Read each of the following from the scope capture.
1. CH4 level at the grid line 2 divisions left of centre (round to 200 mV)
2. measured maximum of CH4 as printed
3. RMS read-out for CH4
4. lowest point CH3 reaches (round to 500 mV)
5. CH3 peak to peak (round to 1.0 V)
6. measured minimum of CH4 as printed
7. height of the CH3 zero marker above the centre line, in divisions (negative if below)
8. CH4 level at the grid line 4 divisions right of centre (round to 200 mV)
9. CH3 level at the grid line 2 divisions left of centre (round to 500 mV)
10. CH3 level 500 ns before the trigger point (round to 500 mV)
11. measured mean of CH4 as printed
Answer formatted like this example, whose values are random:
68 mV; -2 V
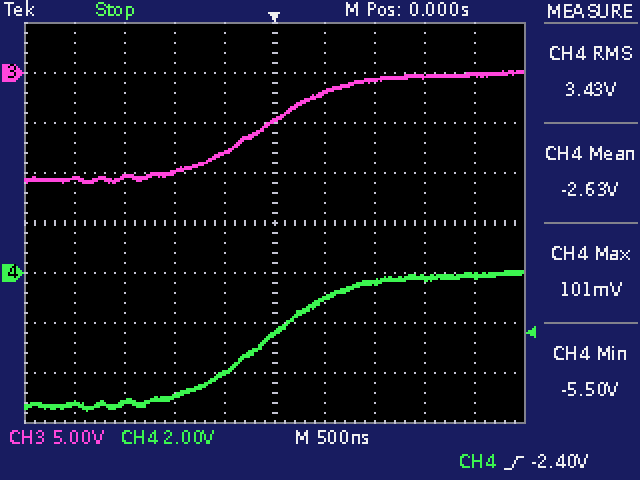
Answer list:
-5.0 V; 101 mV; 3.43 V; -11.0 V; 11.0 V; -5.50 V; +3.0 div; -200 mV; -10.0 V; -8.0 V; -2.63 V
